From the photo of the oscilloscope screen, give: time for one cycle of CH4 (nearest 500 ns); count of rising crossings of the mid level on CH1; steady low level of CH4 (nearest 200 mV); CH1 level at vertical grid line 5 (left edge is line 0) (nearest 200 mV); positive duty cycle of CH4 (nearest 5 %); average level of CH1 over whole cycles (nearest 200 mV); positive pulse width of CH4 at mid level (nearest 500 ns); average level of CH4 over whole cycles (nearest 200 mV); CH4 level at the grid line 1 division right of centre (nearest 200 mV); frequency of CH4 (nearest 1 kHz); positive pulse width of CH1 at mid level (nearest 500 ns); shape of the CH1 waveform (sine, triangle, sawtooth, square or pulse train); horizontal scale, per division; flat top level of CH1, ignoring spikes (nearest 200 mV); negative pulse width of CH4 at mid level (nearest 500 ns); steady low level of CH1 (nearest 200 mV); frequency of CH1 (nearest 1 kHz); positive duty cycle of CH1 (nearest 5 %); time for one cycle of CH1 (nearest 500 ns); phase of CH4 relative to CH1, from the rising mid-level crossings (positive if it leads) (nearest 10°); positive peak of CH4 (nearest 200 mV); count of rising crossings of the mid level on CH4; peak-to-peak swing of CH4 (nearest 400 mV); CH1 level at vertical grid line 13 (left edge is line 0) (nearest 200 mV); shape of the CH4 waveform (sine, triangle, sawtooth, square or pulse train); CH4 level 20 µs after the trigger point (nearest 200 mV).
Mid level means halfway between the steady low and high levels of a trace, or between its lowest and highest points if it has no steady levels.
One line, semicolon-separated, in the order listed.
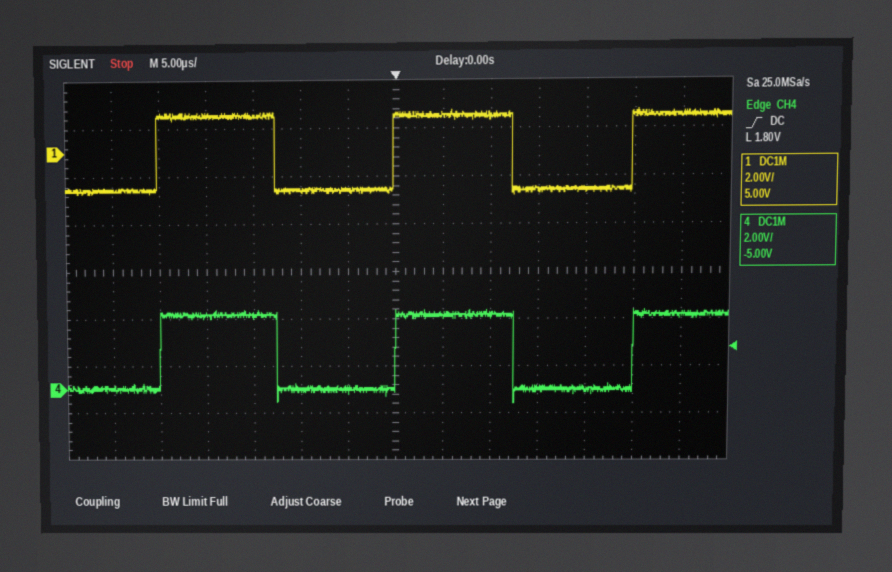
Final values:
25.0 µs; 3; 0.0 V; -1.6 V; 50 %; 0.0 V; 12.5 µs; 1.6 V; 3.2 V; 40 kHz; 12.5 µs; square; 5 µs; 1.6 V; 12.5 µs; -1.6 V; 40 kHz; 50 %; 25.0 µs; 0°; 3.4 V; 3; 4.0 V; 1.6 V; square; 0.0 V
